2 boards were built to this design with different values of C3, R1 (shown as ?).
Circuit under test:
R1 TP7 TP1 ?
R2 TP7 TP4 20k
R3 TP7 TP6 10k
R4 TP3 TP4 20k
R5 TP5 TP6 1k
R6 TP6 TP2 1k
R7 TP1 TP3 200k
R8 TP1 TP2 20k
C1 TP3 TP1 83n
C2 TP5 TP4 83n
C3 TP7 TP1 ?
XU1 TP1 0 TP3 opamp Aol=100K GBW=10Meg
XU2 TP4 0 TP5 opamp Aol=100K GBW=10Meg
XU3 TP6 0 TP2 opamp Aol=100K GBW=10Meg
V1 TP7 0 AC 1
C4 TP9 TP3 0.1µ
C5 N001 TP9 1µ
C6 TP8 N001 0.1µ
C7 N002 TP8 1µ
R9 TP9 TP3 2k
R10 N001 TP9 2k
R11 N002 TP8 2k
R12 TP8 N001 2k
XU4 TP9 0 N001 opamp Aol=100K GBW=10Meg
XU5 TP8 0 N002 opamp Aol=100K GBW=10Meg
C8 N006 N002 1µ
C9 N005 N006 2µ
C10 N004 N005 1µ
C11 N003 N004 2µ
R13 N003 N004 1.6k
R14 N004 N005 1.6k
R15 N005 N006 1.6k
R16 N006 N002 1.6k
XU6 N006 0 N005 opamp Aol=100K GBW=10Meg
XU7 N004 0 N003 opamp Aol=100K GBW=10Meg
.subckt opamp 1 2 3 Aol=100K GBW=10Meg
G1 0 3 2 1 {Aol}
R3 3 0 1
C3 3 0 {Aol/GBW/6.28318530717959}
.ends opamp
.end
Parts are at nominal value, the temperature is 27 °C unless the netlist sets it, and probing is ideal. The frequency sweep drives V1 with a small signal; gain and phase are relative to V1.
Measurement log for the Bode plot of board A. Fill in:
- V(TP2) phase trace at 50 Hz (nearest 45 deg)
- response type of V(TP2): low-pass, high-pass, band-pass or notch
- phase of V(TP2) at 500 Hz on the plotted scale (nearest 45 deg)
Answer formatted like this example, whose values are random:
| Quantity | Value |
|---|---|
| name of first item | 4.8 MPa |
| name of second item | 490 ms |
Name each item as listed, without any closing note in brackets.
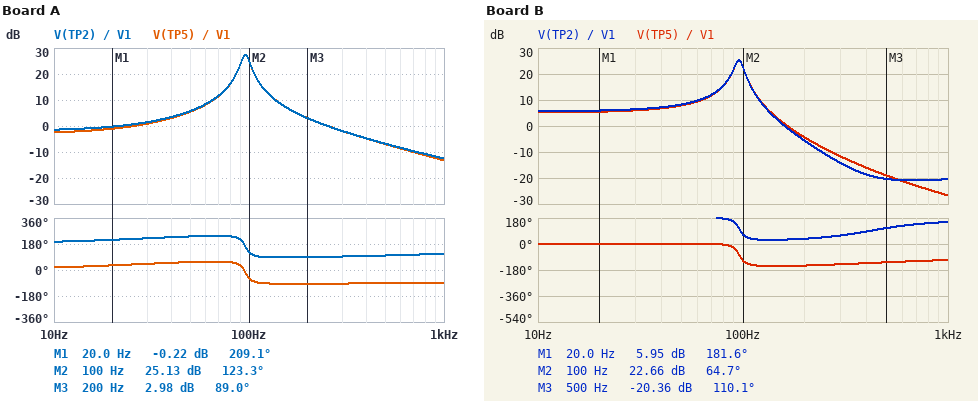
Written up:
| Quantity | Value |
|---|---|
| V(TP2) phase trace at 50 Hz | 225 deg |
| response type of V(TP2): low-pass, high-pass, band-pass or notch | band-pass |
| phase of V(TP2) at 500 Hz on the plotted scale | 90 deg |
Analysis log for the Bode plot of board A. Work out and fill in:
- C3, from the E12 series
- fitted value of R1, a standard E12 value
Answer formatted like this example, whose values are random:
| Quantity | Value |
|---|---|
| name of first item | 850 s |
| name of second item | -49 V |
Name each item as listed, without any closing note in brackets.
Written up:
| Quantity | Value |
|---|---|
| C3, from the E12 series | 270 nF |
| fitted value of R1, a standard E12 value | 22 kΩ |
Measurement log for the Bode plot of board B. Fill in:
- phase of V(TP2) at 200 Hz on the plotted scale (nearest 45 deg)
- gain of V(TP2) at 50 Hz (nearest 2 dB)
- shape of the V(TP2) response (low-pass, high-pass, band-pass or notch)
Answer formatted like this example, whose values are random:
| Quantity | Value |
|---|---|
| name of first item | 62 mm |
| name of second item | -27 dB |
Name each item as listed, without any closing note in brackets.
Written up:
| Quantity | Value |
|---|---|
| phase of V(TP2) at 200 Hz on the plotted scale | 45 deg |
| gain of V(TP2) at 50 Hz | 8 dB |
| shape of the V(TP2) response | band-pass |
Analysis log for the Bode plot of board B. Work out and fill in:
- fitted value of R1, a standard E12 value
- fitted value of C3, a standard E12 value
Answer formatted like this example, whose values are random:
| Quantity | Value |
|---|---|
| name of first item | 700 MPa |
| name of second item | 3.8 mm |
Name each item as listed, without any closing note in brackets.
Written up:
| Quantity | Value |
|---|---|
| fitted value of R1, a standard E12 value | 10 kΩ |
| fitted value of C3, a standard E12 value | 120 nF |
